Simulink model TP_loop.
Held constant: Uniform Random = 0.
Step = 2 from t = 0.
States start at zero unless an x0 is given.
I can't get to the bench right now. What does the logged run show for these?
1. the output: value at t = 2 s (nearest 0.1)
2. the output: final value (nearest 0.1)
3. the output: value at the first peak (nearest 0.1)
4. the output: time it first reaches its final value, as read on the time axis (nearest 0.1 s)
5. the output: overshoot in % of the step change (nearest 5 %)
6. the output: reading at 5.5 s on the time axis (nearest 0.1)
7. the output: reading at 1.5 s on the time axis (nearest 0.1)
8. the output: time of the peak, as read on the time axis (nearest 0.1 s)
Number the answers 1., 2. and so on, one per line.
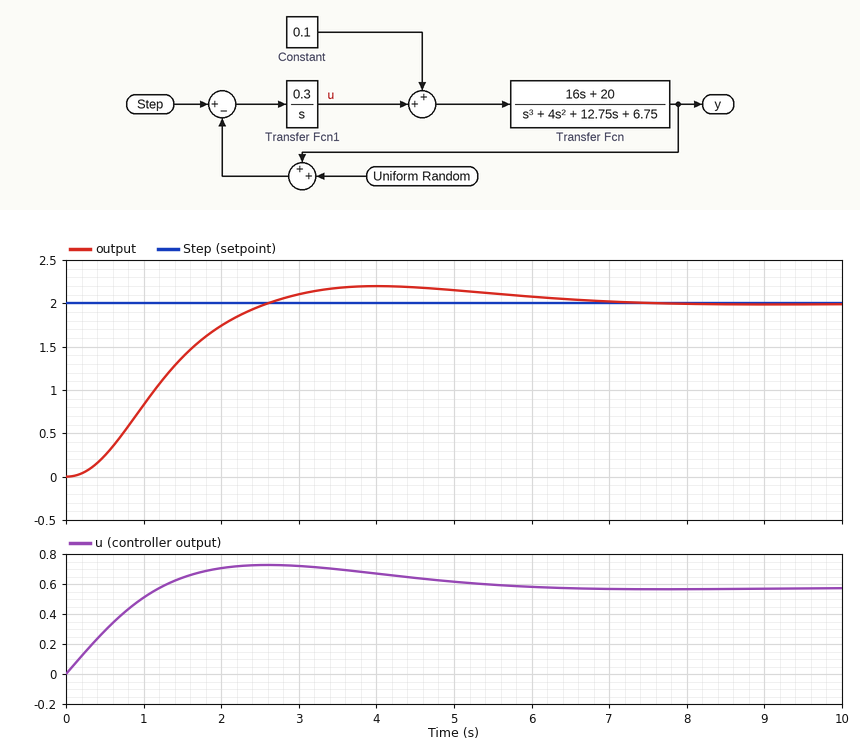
1. 1.7
2. 2.0
3. 2.2
4. 2.6 s
5. 10 %
6. 2.1
7. 1.4
8. 4.0 s
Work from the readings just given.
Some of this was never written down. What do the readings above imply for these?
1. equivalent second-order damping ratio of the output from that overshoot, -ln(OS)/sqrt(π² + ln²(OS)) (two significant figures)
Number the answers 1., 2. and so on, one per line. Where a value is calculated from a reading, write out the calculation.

1. ln(0.1) = -2.303; 2.303 / sqrt(9.870 + 5.302) = 0.59
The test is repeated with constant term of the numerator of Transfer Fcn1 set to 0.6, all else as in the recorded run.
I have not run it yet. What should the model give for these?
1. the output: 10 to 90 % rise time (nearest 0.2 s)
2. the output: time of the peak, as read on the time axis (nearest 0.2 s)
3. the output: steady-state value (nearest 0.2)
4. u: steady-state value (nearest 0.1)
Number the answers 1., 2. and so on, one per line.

1. 0.8 s
2. 2.0 s
3. 2.0
4. 0.6
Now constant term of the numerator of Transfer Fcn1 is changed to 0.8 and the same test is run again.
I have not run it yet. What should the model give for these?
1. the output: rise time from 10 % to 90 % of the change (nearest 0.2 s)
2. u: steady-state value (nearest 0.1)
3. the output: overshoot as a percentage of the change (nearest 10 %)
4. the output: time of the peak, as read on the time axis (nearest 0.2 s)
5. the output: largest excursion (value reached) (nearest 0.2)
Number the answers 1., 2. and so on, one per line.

1. 0.6 s
2. 0.6
3. 40 %
4. 1.8 s
5. 2.8
